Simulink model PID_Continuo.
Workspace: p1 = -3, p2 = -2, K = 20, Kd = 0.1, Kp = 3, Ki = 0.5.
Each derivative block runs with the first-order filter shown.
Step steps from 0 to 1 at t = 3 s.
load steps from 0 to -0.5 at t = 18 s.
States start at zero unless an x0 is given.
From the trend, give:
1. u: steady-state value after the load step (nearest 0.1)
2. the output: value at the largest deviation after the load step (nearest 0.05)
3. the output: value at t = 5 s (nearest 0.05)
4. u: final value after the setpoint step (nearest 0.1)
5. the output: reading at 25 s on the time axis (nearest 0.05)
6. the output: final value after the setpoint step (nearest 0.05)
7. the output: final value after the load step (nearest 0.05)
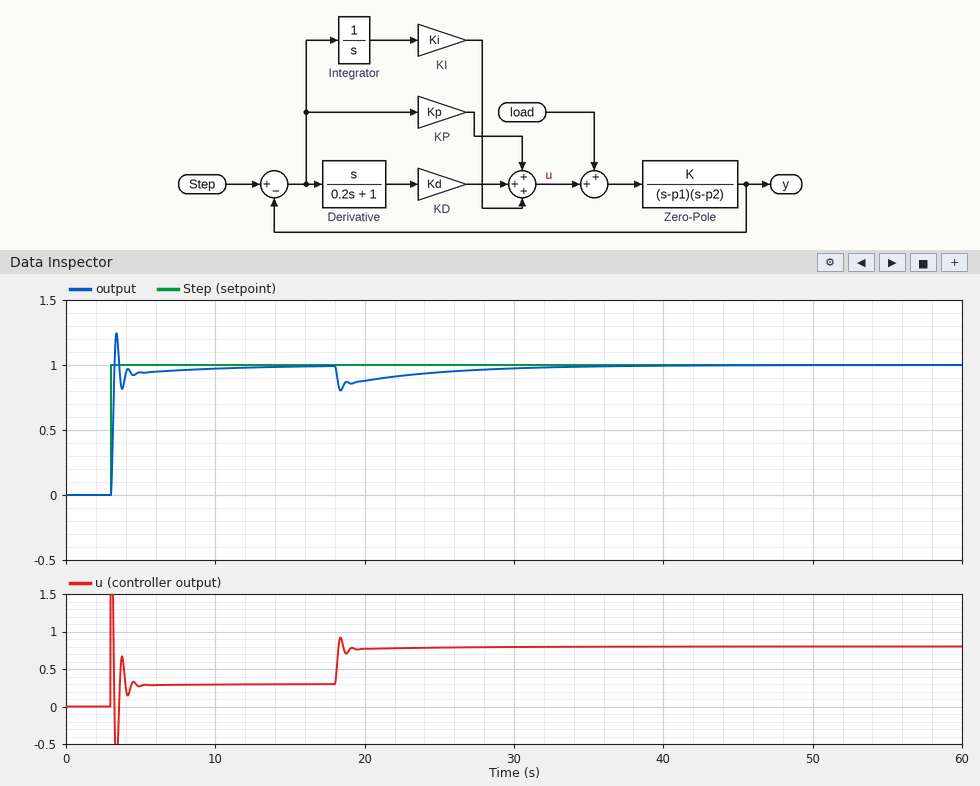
0.8
0.80
0.95
0.3
0.95
1.00
1.00
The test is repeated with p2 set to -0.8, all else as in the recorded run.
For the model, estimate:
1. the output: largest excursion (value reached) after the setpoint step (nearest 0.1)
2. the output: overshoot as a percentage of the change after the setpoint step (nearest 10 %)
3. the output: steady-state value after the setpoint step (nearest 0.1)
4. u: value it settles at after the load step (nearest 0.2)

1.4
40 %
1.0
0.6
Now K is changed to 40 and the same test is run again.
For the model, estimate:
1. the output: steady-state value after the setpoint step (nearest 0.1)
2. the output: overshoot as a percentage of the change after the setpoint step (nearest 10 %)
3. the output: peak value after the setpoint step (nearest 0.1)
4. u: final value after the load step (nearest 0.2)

1.0
40 %
1.4
0.6
